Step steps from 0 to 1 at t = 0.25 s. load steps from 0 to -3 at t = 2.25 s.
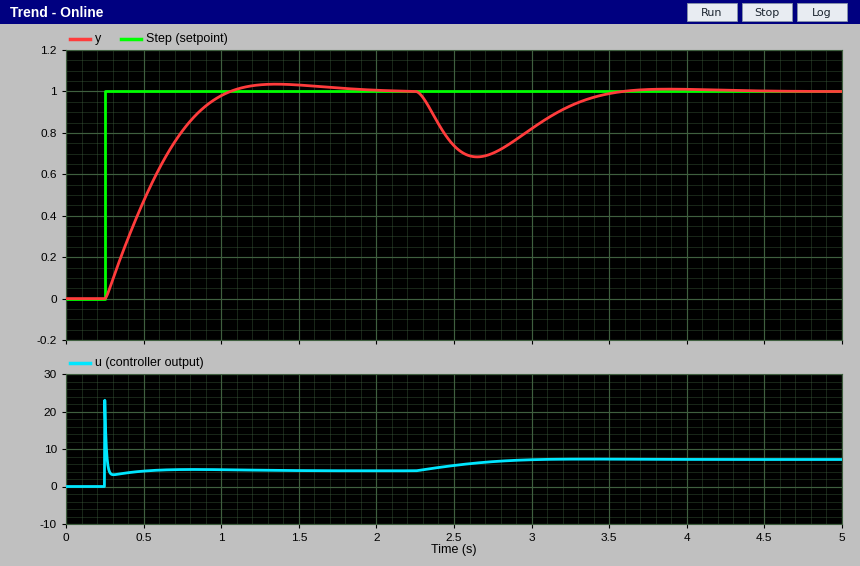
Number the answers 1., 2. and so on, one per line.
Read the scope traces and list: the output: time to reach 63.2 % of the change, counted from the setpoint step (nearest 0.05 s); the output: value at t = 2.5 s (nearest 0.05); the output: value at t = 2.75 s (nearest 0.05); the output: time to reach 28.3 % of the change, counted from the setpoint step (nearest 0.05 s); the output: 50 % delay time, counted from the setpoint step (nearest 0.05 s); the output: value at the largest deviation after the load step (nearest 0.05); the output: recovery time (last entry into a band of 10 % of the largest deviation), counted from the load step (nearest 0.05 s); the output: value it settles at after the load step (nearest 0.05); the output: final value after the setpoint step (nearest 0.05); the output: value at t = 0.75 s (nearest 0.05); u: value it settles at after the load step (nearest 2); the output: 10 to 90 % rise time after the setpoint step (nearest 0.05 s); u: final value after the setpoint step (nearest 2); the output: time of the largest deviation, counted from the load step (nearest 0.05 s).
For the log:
1. 0.35 s
2. 0.75
3. 0.70
4. 0.15 s
5. 0.25 s
6. 0.70
7. 1.15 s
8. 1.00
9. 1.00
10. 0.80
11. 8
12. 0.55 s
13. 4
14. 0.40 s
